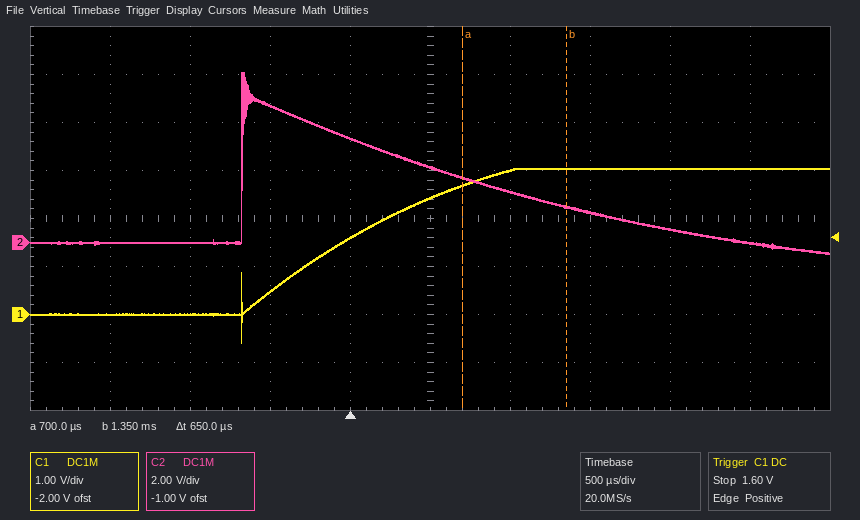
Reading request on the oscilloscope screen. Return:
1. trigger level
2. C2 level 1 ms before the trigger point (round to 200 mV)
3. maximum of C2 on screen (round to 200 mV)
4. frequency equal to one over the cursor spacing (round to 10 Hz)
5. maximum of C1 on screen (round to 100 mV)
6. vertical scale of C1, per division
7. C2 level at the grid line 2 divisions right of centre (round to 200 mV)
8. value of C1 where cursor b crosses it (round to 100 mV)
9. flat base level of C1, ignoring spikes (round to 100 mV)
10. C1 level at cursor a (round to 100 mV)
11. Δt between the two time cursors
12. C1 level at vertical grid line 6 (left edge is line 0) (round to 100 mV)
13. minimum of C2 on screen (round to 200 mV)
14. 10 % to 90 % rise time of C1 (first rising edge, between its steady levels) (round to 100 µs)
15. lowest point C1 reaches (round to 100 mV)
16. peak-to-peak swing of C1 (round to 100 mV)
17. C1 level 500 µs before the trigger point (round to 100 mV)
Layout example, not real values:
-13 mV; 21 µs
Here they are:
1.60 V; 0.0 V; 7.0 V; 1.54 kHz; 3.0 V; 1 V; 1.2 V; 3.0 V; 0.0 V; 2.7 V; 650 µs; 3.0 V; -400 mV; 1.3 ms; -600 mV; 3.6 V; 500 mV
